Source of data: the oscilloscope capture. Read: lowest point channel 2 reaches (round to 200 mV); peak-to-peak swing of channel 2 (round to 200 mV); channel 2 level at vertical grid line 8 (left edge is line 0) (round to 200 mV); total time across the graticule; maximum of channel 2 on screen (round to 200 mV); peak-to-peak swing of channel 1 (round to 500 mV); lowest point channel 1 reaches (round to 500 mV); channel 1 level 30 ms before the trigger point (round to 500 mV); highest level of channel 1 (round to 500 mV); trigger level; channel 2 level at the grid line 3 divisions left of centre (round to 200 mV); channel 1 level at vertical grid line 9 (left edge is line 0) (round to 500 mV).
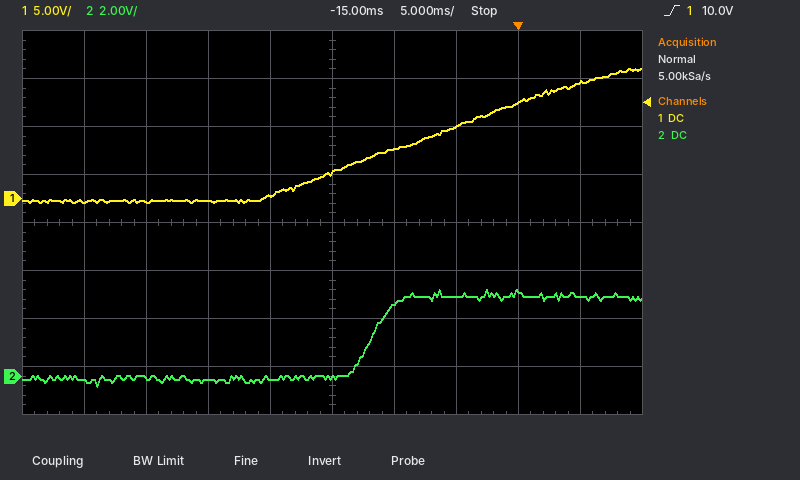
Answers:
-400 mV
4.0 V
3.6 V
50 ms
3.6 V
14.0 V
-500 mV
-500 mV
13.5 V
10.0 V
0.0 V
12.0 V
